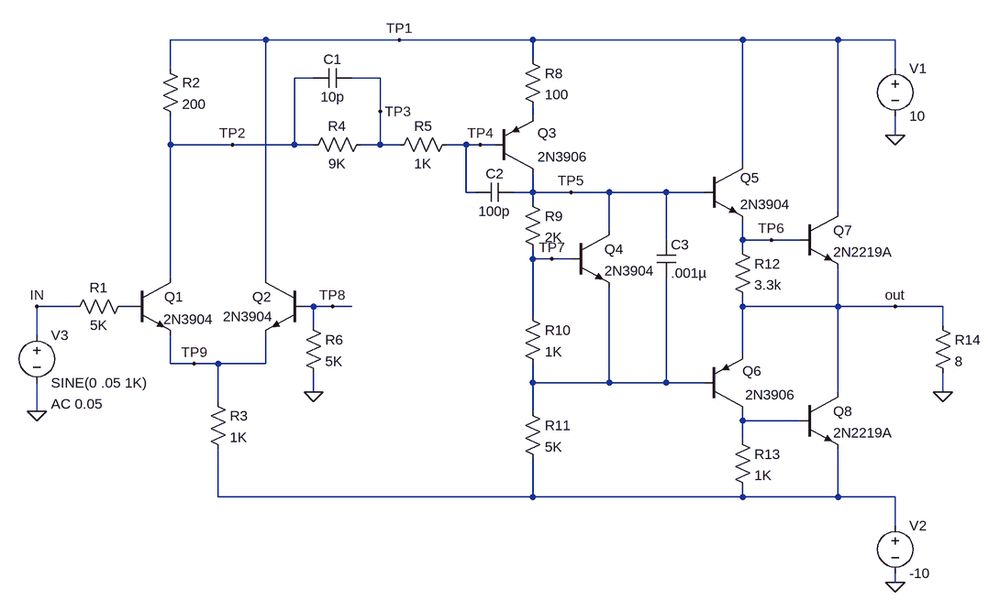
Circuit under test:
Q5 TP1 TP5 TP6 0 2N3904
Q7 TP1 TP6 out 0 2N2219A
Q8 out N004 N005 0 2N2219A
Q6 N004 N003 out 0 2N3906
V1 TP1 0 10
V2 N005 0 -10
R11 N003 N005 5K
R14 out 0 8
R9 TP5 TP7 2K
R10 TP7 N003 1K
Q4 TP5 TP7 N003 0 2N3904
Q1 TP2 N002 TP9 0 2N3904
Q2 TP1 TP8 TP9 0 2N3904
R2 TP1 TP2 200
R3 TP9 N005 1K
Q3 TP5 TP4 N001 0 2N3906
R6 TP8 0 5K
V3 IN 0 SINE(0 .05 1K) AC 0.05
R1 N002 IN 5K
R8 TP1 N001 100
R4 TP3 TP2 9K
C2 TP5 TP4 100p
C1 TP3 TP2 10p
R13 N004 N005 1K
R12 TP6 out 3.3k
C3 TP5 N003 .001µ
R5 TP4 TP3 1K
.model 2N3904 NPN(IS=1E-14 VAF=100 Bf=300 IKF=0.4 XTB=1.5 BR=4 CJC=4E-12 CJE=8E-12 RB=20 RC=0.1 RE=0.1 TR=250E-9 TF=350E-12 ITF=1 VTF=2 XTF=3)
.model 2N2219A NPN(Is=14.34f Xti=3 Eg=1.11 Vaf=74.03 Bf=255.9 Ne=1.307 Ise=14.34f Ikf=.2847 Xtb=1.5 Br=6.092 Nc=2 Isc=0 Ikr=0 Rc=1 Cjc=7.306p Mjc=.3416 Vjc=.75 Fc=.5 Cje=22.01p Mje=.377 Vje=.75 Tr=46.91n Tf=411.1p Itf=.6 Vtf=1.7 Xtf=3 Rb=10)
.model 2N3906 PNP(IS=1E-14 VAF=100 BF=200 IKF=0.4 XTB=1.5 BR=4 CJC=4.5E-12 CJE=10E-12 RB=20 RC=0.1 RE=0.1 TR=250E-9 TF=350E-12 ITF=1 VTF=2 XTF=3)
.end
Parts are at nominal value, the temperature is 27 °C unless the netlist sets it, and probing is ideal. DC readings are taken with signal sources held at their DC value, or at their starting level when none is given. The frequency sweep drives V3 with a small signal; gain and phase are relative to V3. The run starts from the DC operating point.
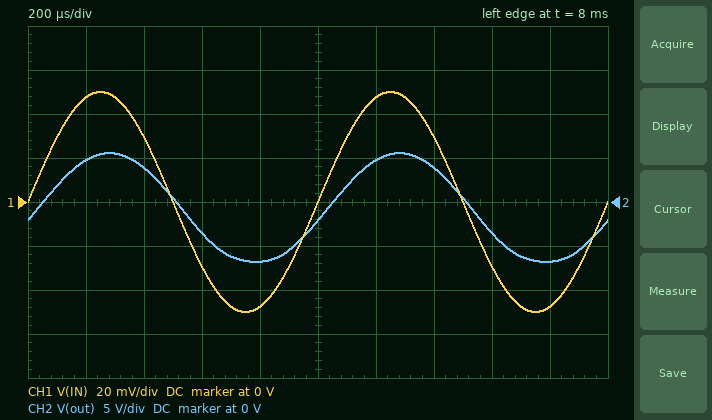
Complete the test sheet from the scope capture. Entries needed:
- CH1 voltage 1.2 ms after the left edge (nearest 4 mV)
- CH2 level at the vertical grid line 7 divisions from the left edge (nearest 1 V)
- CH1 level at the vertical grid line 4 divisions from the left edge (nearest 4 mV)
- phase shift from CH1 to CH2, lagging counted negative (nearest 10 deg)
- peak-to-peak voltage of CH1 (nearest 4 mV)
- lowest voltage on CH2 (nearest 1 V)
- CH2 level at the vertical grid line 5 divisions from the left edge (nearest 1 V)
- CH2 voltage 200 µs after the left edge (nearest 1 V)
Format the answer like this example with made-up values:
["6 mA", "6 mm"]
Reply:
["48 mV", "4 V", "-48 mV", "-10 deg", "100 mV", "-7 V", "-2 V", "5 V"]
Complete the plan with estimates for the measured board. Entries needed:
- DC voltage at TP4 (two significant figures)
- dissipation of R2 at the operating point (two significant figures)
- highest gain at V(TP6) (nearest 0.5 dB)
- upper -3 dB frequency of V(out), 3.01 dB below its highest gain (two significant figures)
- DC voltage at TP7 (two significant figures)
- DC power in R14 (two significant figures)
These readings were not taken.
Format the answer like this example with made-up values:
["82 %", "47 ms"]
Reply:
["9.2 V", "4.2 mW", "43.0 dB", "5.0 kHz", "-850 mV", "88 mW"]
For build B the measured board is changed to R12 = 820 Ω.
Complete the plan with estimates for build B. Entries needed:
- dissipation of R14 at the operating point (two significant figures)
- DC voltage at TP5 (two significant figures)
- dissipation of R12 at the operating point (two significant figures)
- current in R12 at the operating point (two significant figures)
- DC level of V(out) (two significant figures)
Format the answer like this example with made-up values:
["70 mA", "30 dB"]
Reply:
["90 mW", "460 mV", "540 µW", "810 µA", "-850 mV"]
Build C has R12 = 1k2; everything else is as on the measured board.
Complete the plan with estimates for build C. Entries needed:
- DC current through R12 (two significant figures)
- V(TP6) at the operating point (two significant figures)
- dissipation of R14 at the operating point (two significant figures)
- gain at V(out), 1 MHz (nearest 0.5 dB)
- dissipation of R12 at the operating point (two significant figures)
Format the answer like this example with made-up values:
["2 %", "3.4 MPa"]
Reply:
["560 µA", "-170 mV", "89 mW", "-5.0 dB", "380 µW"]
